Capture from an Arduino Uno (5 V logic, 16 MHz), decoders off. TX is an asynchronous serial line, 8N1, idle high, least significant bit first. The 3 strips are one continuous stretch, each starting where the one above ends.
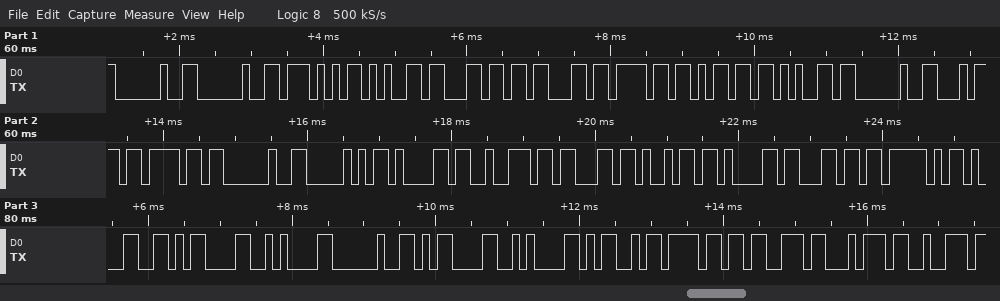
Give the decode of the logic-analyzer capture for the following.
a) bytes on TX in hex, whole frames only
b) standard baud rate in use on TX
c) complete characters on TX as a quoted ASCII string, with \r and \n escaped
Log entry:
0x20 0x20 0x57 0x65 0x6C 0x63 0x6F 0x6D 0x65 0x20 0x74 0x6F 0x20 0x50 0x61 0x72 0x63 0x69 0x61 0x6C 0x5F 0x31 0x0D 0x0A 0x20 0x0D 0x0A 0x4D 0x6F 0x73 0x74 0x72
9600 baud
"  Welcome to Parcial_1\r\n \r\nMostr"
